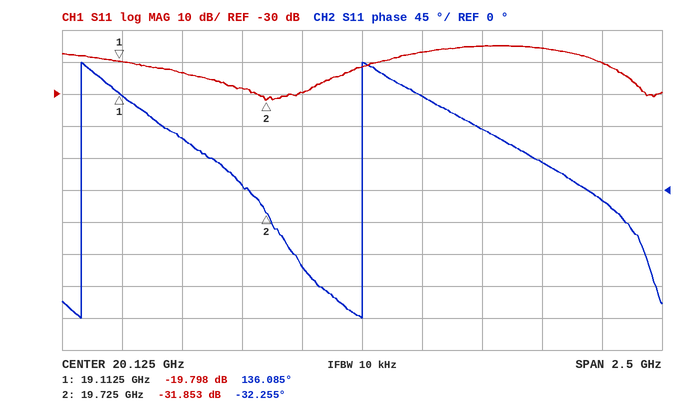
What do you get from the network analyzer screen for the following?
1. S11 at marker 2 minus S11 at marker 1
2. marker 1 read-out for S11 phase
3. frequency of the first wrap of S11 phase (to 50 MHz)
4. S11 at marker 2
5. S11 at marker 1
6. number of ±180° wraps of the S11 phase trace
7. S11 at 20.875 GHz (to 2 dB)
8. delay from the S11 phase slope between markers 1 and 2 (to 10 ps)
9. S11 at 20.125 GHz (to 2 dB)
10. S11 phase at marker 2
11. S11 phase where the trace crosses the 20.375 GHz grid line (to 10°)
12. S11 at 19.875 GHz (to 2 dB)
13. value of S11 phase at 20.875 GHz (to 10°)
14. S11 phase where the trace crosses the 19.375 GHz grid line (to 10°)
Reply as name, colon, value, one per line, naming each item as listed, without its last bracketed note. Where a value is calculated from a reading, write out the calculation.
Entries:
S11 at marker 2 minus S11 at marker 1: -31.853 − (-19.798) = -12.055 dB
marker 1 read-out for S11 phase: 136.085°
frequency of the first wrap of S11 phase: 18.95 GHz
S11 at marker 2: -31.853 dB
S11 at marker 1: -19.798 dB
number of ±180° wraps of the S11 phase trace: 2
S11 at 20.875 GHz: -16 dB
delay from the S11 phase slope between markers 1 and 2: −(-32.255° − (136.085°))/(360° × 612.5 MHz) ≈ 763 ps, so 760 ps to the nearest 10 ps
S11 at 20.125 GHz: -22 dB
S11 phase at marker 2: -32.255°
S11 phase where the trace crosses the 20.375 GHz grid line: 130°
S11 at 19.875 GHz: -30 dB
value of S11 phase at 20.875 GHz: 40°
S11 phase where the trace crosses the 19.375 GHz grid line: 70°
